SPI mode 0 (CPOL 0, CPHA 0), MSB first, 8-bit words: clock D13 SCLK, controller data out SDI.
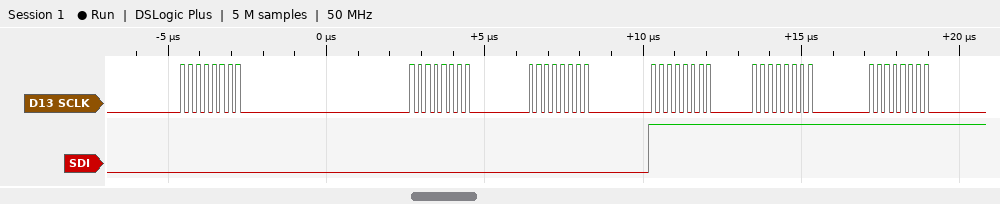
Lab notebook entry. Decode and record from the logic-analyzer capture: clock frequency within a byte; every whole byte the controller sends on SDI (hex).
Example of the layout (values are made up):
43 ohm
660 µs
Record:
4 MHz
0x00 0x00 0x00 0xFF 0xFF 0xFF
